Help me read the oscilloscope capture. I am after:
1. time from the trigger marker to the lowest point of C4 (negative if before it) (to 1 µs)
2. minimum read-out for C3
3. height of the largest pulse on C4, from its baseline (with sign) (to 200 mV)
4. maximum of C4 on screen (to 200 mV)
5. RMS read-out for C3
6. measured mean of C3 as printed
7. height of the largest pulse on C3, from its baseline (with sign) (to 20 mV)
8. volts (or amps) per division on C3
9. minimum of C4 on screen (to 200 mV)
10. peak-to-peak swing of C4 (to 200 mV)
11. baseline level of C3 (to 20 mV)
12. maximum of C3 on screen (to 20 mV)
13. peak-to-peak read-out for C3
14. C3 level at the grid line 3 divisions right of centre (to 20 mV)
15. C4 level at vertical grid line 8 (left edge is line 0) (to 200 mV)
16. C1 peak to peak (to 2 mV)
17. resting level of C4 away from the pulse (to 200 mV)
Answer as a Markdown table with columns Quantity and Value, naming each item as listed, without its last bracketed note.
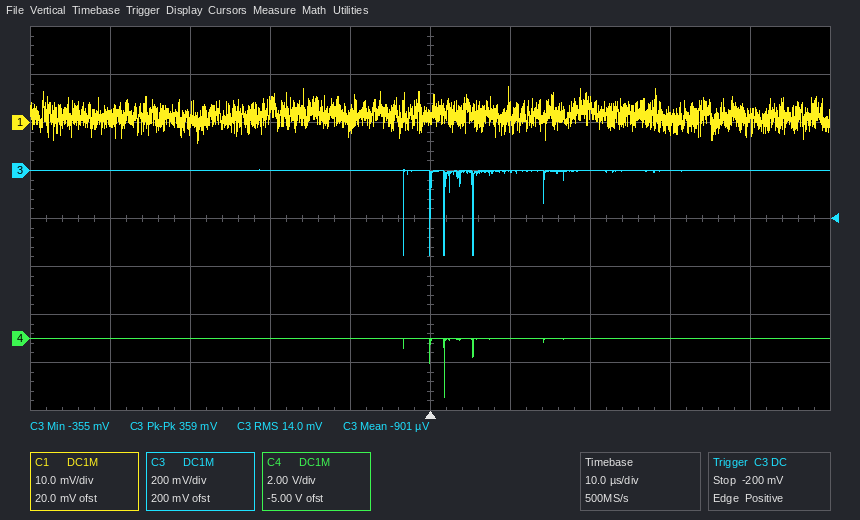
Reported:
| Quantity | Value |
|---|---|
| time from the trigger marker to the lowest point of C4 (negative if before it) | +2 µs |
| minimum read-out for C3 | -355 mV |
| height of the largest pulse on C4, from its baseline (with sign) | -2.4 V |
| maximum of C4 on screen | 0.0 V |
| RMS read-out for C3 | 14.0 mV |
| measured mean of C3 as printed | -901 µV |
| height of the largest pulse on C3, from its baseline (with sign) | -360 mV |
| volts (or amps) per division on C3 | 200 mV |
| minimum of C4 on screen | -2.4 V |
| peak-to-peak swing of C4 | 2.4 V |
| baseline level of C3 | 0 mV |
| maximum of C3 on screen | 0 mV |
| peak-to-peak read-out for C3 | 359 mV |
| C3 level at the grid line 3 divisions right of centre | 0 mV |
| C4 level at vertical grid line 8 (left edge is line 0) | 0.0 V |
| C1 peak to peak | 12 mV |
| resting level of C4 away from the pulse | 0.0 V |
